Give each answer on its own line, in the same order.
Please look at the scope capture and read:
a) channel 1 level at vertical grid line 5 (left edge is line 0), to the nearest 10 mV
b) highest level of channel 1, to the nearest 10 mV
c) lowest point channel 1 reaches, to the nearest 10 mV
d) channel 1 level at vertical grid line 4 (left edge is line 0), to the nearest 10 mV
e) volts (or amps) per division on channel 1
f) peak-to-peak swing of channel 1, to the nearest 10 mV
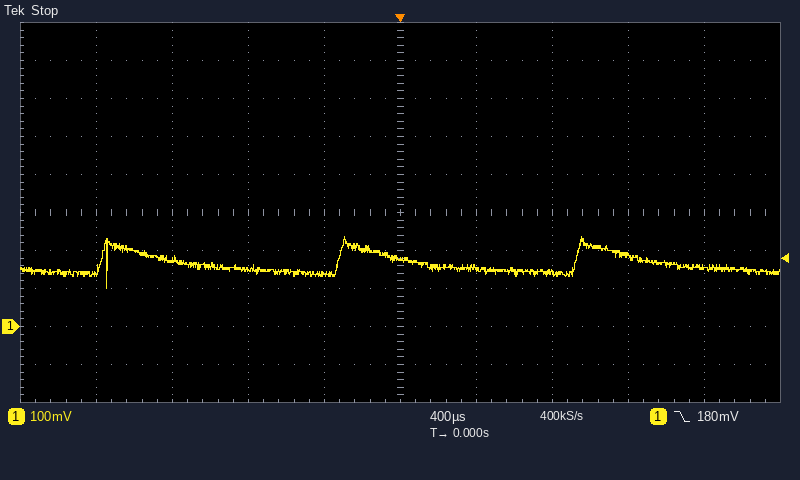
180 mV
240 mV
100 mV
140 mV
100 mV
140 mV
